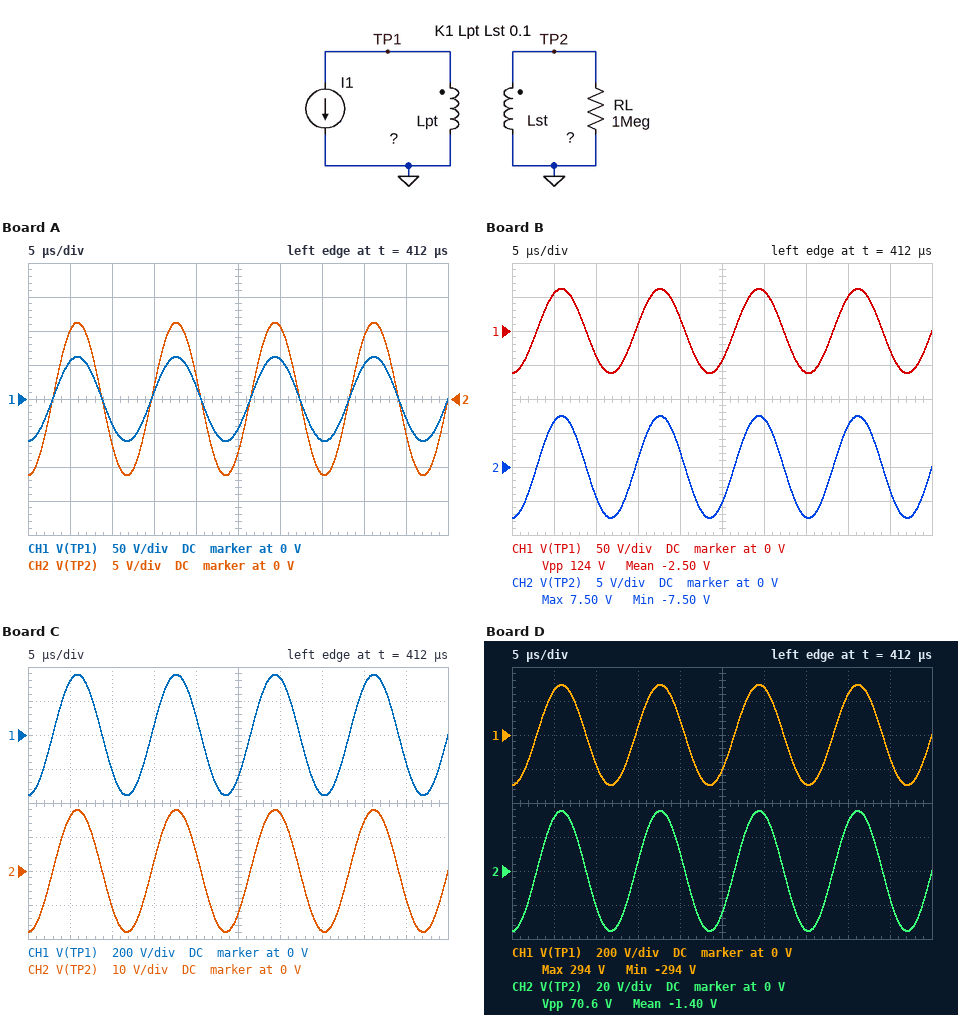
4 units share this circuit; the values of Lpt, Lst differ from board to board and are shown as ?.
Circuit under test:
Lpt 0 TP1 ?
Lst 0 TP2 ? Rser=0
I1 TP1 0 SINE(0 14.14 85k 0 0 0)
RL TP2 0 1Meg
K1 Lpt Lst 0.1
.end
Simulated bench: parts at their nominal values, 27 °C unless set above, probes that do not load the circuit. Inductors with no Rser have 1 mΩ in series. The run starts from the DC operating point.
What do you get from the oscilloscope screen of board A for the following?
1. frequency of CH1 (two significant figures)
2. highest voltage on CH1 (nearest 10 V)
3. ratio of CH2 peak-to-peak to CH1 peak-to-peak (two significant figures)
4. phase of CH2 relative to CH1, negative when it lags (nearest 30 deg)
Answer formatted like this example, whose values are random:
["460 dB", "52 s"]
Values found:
["85 kHz", "60 V", "0.18", "0 deg"]
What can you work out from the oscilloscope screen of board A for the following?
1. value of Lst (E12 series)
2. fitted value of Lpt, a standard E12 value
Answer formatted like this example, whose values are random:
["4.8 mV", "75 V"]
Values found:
["27 µH", "8.2 µH"]
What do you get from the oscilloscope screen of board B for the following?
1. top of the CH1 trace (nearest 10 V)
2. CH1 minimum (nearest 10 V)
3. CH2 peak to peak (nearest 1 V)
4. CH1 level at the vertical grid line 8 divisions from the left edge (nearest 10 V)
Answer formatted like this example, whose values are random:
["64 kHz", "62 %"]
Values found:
["60 V", "-60 V", "15 V", "50 V"]
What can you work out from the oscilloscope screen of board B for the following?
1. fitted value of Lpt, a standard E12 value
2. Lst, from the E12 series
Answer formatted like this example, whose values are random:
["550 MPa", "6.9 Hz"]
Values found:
["8.2 µH", "12 µH"]
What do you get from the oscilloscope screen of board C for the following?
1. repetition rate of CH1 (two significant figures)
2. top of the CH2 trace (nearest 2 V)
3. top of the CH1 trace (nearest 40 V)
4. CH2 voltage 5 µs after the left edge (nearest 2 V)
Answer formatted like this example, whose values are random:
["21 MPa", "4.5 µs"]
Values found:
["85 kHz", "18 V", "360 V", "16 V"]
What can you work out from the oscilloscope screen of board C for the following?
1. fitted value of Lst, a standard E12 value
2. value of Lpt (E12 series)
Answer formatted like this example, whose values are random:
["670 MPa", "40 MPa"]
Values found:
["12 µH", "47 µH"]
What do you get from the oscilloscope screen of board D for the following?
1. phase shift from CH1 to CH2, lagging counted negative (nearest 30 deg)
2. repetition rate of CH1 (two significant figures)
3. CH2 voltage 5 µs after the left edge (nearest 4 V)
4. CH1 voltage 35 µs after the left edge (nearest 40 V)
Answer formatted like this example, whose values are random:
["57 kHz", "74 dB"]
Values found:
["0 deg", "85 kHz", "32 V", "-280 V"]
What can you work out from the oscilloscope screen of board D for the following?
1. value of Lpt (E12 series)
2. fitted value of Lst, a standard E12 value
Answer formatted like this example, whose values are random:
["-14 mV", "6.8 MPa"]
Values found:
["39 µH", "56 µH"]
